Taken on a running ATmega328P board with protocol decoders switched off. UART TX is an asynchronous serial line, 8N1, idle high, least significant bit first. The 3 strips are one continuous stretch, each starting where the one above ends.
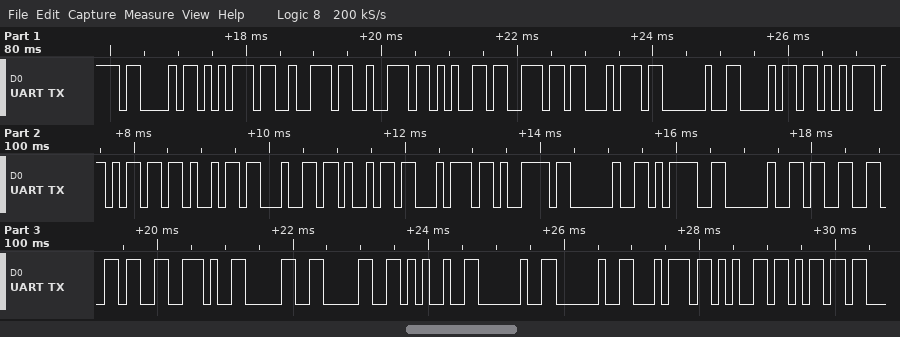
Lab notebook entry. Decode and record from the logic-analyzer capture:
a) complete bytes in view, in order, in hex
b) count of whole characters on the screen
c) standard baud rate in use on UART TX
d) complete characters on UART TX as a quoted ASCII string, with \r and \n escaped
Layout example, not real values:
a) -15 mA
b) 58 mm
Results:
a) 43 75 72 72 65 6E 74 20 68 75 6D 69 64 69 74 79 20 3D 20 33 36 2E 30 30 25 20 20 74 65 6D
b) 30
c) 9600 baud
d) "Current humidity = 36.00%  tem"
